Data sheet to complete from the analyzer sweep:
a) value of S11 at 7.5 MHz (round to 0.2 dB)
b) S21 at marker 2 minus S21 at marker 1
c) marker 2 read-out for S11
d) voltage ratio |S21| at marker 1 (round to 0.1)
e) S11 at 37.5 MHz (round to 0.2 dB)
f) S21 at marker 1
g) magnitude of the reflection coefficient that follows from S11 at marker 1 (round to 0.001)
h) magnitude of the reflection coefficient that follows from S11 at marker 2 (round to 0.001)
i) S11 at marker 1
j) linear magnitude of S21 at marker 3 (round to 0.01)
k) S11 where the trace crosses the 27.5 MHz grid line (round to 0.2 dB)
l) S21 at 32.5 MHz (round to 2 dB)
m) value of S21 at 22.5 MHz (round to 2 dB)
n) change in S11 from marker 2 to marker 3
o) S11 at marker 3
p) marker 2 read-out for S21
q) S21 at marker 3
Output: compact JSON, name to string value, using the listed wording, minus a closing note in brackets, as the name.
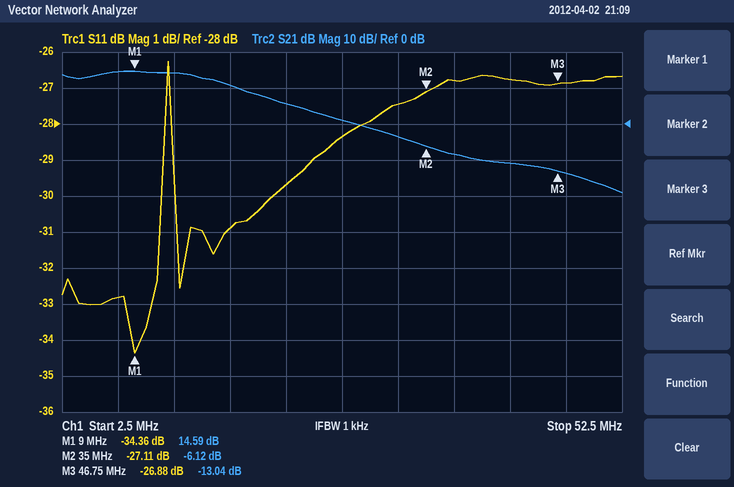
{"value of S11 at 7.5 MHz": "-32.8 dB", "S21 at marker 2 minus S21 at marker 1": "-20.71 dB", "marker 2 read-out for S11": "-27.11 dB", "voltage ratio |S21| at marker 1": "5.4", "S11 at 37.5 MHz": "-26.8 dB", "S21 at marker 1": "14.59 dB", "magnitude of the reflection coefficient that follows from S11 at marker 1": "0.019", "magnitude of the reflection coefficient that follows from S11 at marker 2": "0.044", "S11 at marker 1": "-34.36 dB", "linear magnitude of S21 at marker 3": "0.22", "S11 where the trace crosses the 27.5 MHz grid line": "-28.4 dB", "S21 at 32.5 MHz": "-4 dB", "value of S21 at 22.5 MHz": "6 dB", "change in S11 from marker 2 to marker 3": "0.23 dB", "S11 at marker 3": "-26.88 dB", "marker 2 read-out for S21": "-6.12 dB", "S21 at marker 3": "-13.04 dB"}
